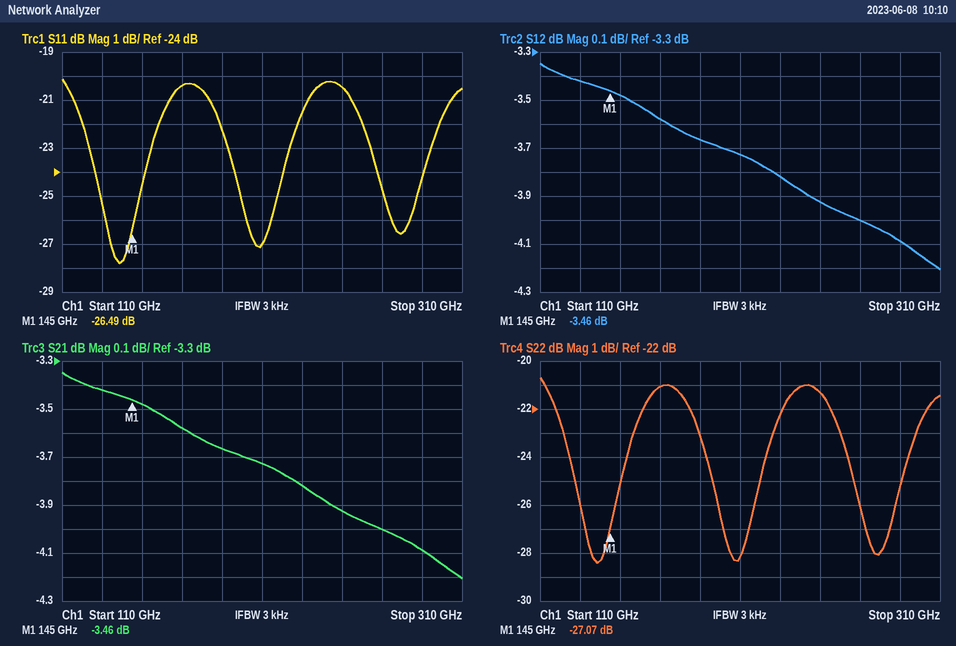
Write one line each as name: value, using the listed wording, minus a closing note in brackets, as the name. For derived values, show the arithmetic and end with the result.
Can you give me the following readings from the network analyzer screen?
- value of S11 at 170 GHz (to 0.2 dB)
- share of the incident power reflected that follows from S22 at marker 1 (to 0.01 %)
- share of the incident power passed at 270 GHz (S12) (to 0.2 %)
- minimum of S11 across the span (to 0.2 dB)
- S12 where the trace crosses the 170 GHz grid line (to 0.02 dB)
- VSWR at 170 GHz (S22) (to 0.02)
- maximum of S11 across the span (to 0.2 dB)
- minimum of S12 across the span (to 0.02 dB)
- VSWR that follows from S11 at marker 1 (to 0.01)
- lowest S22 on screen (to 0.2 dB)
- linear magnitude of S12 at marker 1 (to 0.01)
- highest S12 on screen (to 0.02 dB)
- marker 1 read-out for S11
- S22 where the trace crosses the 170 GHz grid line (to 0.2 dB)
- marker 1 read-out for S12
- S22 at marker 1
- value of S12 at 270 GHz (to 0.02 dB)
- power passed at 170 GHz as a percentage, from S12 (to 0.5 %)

value of S11 at 170 GHz: -20.4 dB
share of the incident power reflected that follows from S22 at marker 1: 10^(-27.07/10) ≈ 0.20 %
share of the incident power passed at 270 GHz (S12): 10^(-4/10) ≈ 39.8 %
minimum of S11 across the span: -27.8 dB
S12 where the trace crosses the 170 GHz grid line: -3.58 dB
VSWR at 170 GHz (S22): |Γ| = 10^(-21/20) = 0.0891; VSWR = (1 + 0.0891)/(1 − 0.0891) ≈ 1.20
maximum of S11 across the span: -20.2 dB
minimum of S12 across the span: -4.20 dB
VSWR that follows from S11 at marker 1: (1 + 0.0474)/(1 − 0.0474) ≈ 1.10
lowest S22 on screen: -28.4 dB
linear magnitude of S12 at marker 1: 10^(-3.46/20) ≈ 0.67
highest S12 on screen: -3.34 dB
marker 1 read-out for S11: -26.49 dB
S22 where the trace crosses the 170 GHz grid line: -21.0 dB
marker 1 read-out for S12: -3.46 dB
S22 at marker 1: -27.07 dB
value of S12 at 270 GHz: -4.00 dB
power passed at 170 GHz as a percentage, from S12: 10^(-3.58/10) ≈ 43.9 %, so 44.0 % to the nearest 0.5 %
